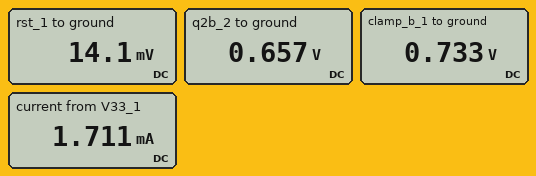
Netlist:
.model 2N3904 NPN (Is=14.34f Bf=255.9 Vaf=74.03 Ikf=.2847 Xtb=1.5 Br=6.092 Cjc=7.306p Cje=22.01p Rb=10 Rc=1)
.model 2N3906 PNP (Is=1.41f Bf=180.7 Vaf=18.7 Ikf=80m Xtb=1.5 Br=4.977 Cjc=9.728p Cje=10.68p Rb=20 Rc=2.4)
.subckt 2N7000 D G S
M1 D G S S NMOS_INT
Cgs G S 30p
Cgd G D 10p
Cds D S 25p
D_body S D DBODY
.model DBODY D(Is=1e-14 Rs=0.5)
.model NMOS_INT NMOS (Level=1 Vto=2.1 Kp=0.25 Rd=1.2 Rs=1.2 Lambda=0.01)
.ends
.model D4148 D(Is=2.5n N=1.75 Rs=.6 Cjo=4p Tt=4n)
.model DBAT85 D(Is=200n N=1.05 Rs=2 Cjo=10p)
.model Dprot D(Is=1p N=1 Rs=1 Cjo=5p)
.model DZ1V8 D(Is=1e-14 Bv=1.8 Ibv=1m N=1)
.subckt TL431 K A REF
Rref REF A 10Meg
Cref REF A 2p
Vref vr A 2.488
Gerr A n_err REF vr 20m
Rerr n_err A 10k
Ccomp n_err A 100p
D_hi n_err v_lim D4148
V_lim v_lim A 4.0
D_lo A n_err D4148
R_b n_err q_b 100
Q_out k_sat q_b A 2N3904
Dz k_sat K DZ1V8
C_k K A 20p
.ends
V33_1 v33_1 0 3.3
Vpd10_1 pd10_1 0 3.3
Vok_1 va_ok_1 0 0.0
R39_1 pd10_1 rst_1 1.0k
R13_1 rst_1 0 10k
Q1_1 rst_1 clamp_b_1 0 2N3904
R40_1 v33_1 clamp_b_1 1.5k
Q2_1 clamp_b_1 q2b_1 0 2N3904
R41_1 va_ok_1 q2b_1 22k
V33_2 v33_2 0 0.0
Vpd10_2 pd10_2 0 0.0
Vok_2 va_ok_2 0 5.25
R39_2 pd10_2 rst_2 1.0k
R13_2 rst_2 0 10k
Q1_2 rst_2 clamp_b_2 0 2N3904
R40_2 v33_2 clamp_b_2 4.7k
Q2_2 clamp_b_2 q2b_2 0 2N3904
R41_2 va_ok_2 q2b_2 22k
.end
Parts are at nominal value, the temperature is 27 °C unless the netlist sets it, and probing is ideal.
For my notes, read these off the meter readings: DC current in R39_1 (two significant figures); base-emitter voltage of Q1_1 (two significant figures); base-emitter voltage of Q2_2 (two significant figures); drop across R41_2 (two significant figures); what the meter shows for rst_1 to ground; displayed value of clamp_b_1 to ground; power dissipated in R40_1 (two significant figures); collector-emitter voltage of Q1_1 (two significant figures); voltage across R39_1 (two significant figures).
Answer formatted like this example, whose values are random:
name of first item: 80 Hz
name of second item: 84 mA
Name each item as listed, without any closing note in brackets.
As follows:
DC current in R39_1: 3.3 mA
base-emitter voltage of Q1_1: 730 mV
base-emitter voltage of Q2_2: 660 mV
drop across R41_2: 4.6 V
what the meter shows for rst_1 to ground: 14.1 mV
displayed value of clamp_b_1 to ground: 0.733 V
power dissipated in R40_1: 4.4 mW
collector-emitter voltage of Q1_1: 14 mV
voltage across R39_1: 3.3 V
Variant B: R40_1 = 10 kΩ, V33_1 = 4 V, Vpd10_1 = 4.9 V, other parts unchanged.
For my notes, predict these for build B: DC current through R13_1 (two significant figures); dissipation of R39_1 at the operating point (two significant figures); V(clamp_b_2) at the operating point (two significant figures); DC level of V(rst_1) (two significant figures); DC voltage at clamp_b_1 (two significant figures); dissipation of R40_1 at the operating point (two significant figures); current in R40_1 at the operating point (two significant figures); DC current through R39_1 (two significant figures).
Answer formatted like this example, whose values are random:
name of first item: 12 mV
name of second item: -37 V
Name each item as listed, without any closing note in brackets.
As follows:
DC current through R13_1: 4.0 µA
dissipation of R39_1 at the operating point: 24 mW
V(clamp_b_2) at the operating point: 4.0 mV
DC level of V(rst_1): 40 mV
DC voltage at clamp_b_1: 700 mV
dissipation of R40_1 at the operating point: 1.1 mW
current in R40_1 at the operating point: 330 µA
DC current through R39_1: 4.9 mA
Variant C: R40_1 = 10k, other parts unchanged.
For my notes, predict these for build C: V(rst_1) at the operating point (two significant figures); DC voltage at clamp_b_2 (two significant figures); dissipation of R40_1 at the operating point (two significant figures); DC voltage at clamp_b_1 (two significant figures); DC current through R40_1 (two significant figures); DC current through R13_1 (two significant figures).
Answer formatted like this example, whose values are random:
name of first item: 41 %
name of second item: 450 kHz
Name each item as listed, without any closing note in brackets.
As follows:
V(rst_1) at the operating point: 35 mV
DC voltage at clamp_b_2: 4.0 mV
dissipation of R40_1 at the operating point: 680 µW
DC voltage at clamp_b_1: 690 mV
DC current through R40_1: 260 µA
DC current through R13_1: 3.5 µA
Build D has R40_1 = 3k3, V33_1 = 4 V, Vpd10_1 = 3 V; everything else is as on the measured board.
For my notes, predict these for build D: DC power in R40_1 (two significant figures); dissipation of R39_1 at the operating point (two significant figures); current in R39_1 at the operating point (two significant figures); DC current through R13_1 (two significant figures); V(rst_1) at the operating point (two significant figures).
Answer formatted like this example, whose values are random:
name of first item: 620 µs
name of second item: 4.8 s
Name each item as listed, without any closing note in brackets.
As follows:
DC power in R40_1: 3.3 mW
dissipation of R39_1 at the operating point: 8.9 mW
current in R39_1 at the operating point: 3.0 mA
DC current through R13_1: 1.7 µA
V(rst_1) at the operating point: 17 mV
